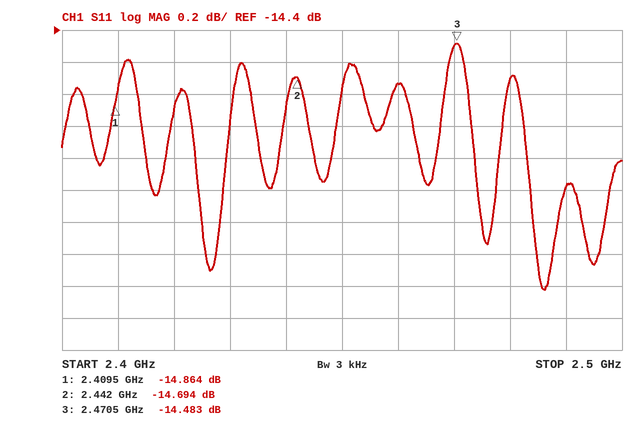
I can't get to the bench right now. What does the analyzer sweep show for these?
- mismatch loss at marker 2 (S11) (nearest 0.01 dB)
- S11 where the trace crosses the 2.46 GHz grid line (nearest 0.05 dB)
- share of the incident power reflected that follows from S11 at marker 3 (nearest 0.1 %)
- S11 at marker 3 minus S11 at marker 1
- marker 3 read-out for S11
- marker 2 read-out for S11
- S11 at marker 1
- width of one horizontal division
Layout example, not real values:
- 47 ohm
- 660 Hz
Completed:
- 0.15 dB
- -14.75 dB
- 3.6 %
- 0.381 dB
- -14.483 dB
- -14.694 dB
- -14.864 dB
- 10 MHz
